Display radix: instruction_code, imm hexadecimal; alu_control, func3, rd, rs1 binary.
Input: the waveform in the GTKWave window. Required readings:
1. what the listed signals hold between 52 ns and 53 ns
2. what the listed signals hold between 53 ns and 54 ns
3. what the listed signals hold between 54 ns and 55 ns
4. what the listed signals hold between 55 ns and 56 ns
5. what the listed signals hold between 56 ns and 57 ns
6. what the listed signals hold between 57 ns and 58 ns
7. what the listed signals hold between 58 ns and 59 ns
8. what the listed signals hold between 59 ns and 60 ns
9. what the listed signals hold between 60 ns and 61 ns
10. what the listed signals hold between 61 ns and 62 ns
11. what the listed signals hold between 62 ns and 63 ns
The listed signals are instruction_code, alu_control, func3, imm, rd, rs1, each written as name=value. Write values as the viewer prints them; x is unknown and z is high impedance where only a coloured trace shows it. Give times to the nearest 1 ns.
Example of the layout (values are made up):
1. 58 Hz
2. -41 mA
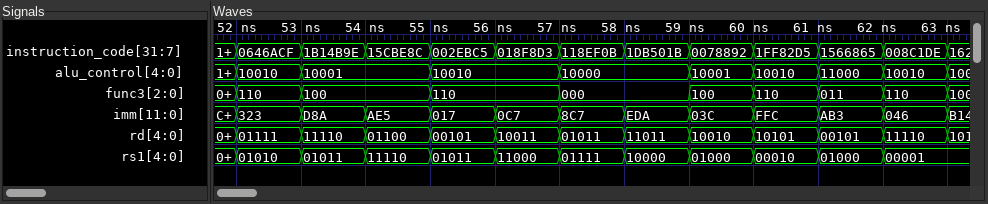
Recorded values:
1. instruction_code=0646ACF, alu_control=10010, func3=110, imm=323, rd=01111, rs1=01010
2. instruction_code=1B14B9E, alu_control=10001, func3=100, imm=D8A, rd=11110, rs1=01011
3. instruction_code=15CBE8C, alu_control=10001, func3=100, imm=AE5, rd=01100, rs1=11110
4. instruction_code=002EBC5, alu_control=10010, func3=110, imm=017, rd=00101, rs1=01011
5. instruction_code=018F8D3, alu_control=10010, func3=110, imm=0C7, rd=10011, rs1=11000
6. instruction_code=118EF0B, alu_control=10000, func3=000, imm=8C7, rd=01011, rs1=01111
7. instruction_code=1DB501B, alu_control=10000, func3=000, imm=EDA, rd=11011, rs1=10000
8. instruction_code=0078892, alu_control=10001, func3=100, imm=03C, rd=10010, rs1=01000
9. instruction_code=1FF82D5, alu_control=10010, func3=110, imm=FFC, rd=10101, rs1=00010
10. instruction_code=1566865, alu_control=11000, func3=011, imm=AB3, rd=00101, rs1=01000
11. instruction_code=008C1DE, alu_control=10010, func3=110, imm=046, rd=11110, rs1=00001
